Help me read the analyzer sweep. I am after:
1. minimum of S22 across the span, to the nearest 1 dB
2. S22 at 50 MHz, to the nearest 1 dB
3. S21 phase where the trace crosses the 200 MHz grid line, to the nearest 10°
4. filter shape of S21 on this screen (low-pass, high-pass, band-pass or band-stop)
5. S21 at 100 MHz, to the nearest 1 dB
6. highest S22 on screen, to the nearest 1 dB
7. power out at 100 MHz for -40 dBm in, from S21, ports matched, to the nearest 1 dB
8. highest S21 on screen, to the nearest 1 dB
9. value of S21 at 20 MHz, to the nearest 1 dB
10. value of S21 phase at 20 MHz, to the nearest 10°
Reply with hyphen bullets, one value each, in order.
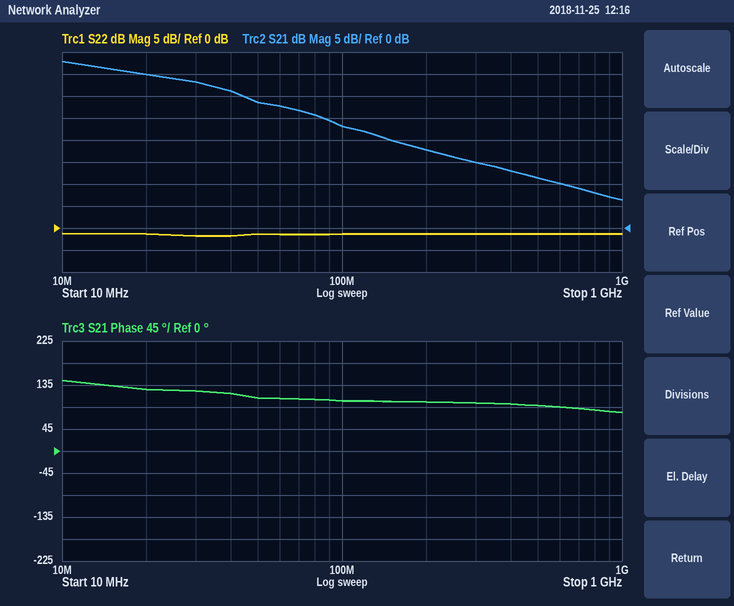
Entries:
- -2 dB
- -1 dB
- 100°
- low-pass
- 23 dB
- -1 dB
- -17 dBm
- 38 dB
- 35 dB
- 130°
